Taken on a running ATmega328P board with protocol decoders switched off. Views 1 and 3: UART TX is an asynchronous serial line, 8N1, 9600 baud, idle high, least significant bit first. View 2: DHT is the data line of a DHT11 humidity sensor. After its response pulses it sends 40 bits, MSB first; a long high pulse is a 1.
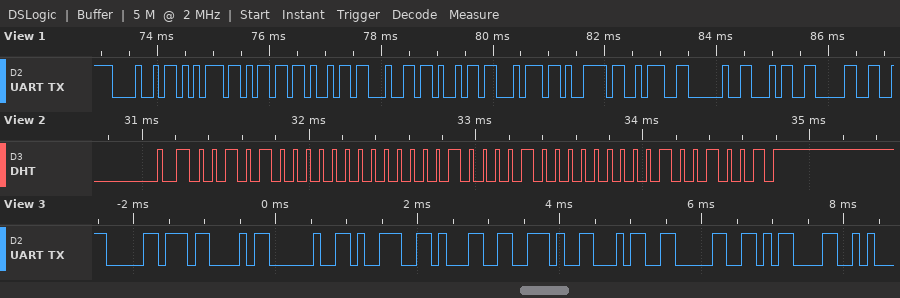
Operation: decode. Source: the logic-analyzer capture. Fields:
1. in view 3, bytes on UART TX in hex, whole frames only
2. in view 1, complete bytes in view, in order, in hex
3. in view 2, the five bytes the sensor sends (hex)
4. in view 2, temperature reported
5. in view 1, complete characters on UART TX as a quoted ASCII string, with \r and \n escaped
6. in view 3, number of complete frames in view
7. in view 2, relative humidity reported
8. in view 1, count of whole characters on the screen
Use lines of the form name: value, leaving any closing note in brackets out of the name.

in view 3, bytes on UART TX in hex, whole frames only: 0xB0 0x43 0x20 0x39 0x31 0x2E 0x34 0x30 0x0D
in view 1, complete bytes in view, in order, in hex: 0x48 0x75 0x6D 0x69 0x64 0x69 0x74 0x79 0x3A 0x20 0x34 0x30
in view 2, the five bytes the sensor sends: 28 00 21 00 49
in view 2, temperature reported: 33.0 °C
in view 1, complete characters on UART TX as a quoted ASCII string, with \r and \n escaped: "Humidity: 40"
in view 3, number of complete frames in view: 9
in view 2, relative humidity reported: 40 %
in view 1, count of whole characters on the screen: 12
